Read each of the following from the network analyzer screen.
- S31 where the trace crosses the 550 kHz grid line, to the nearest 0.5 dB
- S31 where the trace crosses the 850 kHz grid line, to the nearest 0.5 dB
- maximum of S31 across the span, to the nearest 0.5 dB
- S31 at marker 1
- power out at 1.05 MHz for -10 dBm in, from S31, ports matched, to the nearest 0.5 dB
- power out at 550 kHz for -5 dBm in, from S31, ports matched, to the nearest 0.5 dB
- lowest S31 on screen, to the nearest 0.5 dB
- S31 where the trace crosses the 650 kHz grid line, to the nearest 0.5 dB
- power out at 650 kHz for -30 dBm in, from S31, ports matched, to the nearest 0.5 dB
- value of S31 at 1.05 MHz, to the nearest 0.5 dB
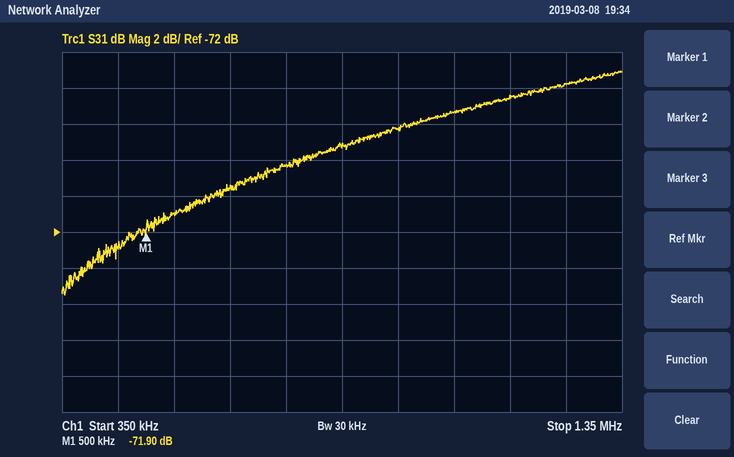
-71.0 dB
-67.0 dB
-63.0 dB
-71.90 dB
-75.5 dBm
-76.0 dBm
-75.5 dB
-69.5 dB
-99.5 dBm
-65.5 dB
